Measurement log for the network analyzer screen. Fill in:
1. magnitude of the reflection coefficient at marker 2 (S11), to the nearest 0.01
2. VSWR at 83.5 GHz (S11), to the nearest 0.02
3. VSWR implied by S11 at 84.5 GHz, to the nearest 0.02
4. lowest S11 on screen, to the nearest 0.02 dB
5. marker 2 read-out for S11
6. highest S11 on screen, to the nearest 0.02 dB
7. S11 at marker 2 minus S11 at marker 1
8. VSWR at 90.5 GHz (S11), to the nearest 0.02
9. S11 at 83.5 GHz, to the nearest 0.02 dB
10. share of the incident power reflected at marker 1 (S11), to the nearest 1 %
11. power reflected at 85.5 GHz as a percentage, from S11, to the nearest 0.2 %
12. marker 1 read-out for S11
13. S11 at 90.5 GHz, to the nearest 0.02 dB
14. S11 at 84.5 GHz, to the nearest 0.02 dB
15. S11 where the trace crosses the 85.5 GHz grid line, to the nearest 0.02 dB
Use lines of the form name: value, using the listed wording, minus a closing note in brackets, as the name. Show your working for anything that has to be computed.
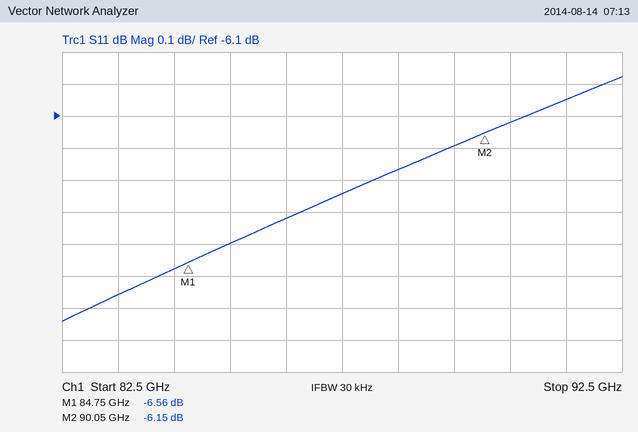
magnitude of the reflection coefficient at marker 2 (S11), to the nearest 0.01: 10^(-6.15/20) ≈ 0.49
VSWR at 83.5 GHz (S11), to the nearest 0.02: |Γ| = 10^(-6.66/20) = 0.4645; VSWR = (1 + 0.4645)/(1 − 0.4645) ≈ 2.73, so 2.74 to the nearest 0.02
VSWR implied by S11 at 84.5 GHz, to the nearest 0.02: |Γ| = 10^(-6.58/20) = 0.4688; VSWR = (1 + 0.4688)/(1 − 0.4688) ≈ 2.77, so 2.76 to the nearest 0.02
lowest S11 on screen, to the nearest 0.02 dB: -6.74 dB
marker 2 read-out for S11: -6.15 dB
highest S11 on screen, to the nearest 0.02 dB: -5.98 dB
S11 at marker 2 minus S11 at marker 1: -6.15 − (-6.56) = 0.41 dB
VSWR at 90.5 GHz (S11), to the nearest 0.02: |Γ| = 10^(-6.12/20) = 0.4943; VSWR = (1 + 0.4943)/(1 − 0.4943) ≈ 2.95, so 2.96 to the nearest 0.02
S11 at 83.5 GHz, to the nearest 0.02 dB: -6.66 dB
share of the incident power reflected at marker 1 (S11), to the nearest 1 %: 10^(-6.56/10) ≈ 22 %
power reflected at 85.5 GHz as a percentage, from S11, to the nearest 0.2 %: 10^(-6.5/10) ≈ 22.4 %
marker 1 read-out for S11: -6.56 dB
S11 at 90.5 GHz, to the nearest 0.02 dB: -6.12 dB
S11 at 84.5 GHz, to the nearest 0.02 dB: -6.58 dB
S11 where the trace crosses the 85.5 GHz grid line, to the nearest 0.02 dB: -6.50 dB
